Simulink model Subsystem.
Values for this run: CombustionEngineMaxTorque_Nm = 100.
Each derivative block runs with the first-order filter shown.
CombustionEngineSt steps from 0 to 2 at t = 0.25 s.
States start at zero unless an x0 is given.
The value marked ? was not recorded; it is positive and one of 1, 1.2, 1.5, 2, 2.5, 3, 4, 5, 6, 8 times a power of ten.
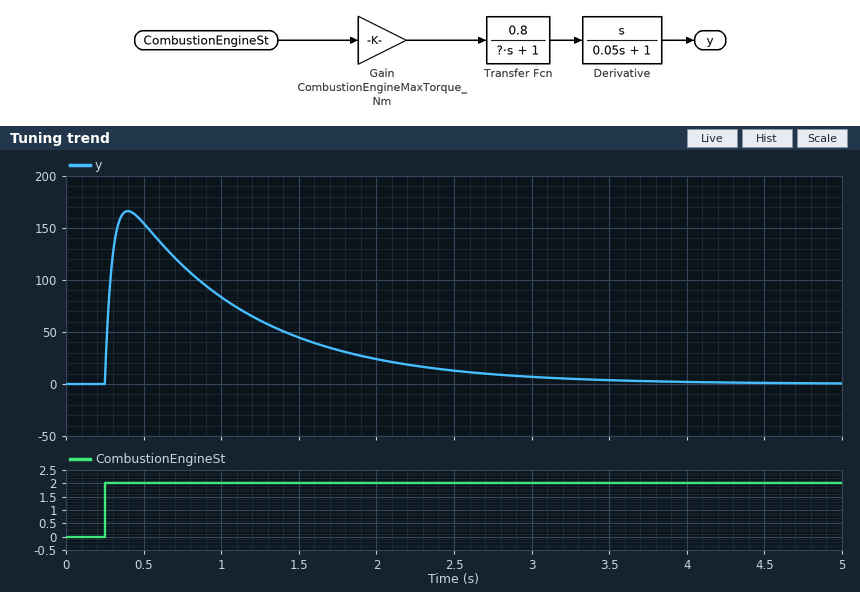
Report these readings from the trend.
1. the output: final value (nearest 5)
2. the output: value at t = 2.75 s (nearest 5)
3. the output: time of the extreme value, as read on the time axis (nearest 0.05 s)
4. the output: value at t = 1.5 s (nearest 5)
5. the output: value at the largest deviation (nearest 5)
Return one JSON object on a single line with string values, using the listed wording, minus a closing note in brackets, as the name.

{"the output: final value": "0", "the output: value at t = 2.75 s": "10", "the output: time of the extreme value, as read on the time axis": "0.40 s", "the output: value at t = 1.5 s": "45", "the output: value at the largest deviation": "165"}
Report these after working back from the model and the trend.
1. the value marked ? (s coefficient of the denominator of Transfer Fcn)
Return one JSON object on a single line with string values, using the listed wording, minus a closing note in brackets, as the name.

{"the value marked ?": "0.8"}
